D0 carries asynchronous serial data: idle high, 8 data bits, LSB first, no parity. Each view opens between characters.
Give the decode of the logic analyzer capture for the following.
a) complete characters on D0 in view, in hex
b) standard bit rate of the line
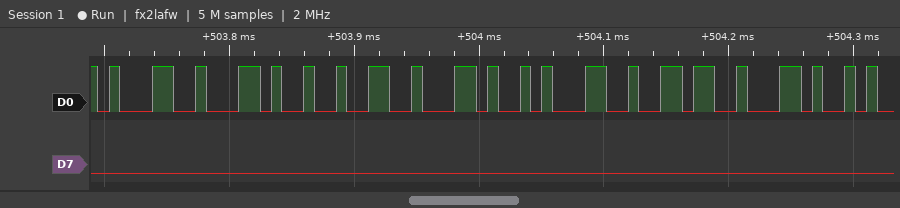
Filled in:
31, 2C, 32, 2C, 31, 36, 2C
115200 baud
